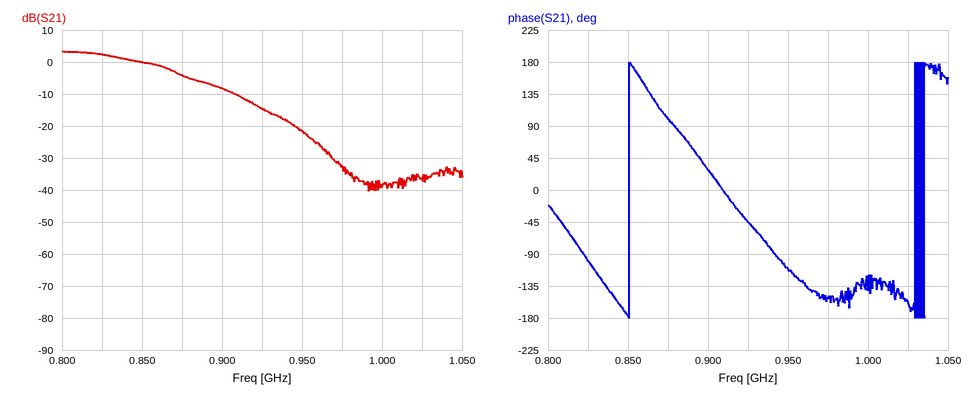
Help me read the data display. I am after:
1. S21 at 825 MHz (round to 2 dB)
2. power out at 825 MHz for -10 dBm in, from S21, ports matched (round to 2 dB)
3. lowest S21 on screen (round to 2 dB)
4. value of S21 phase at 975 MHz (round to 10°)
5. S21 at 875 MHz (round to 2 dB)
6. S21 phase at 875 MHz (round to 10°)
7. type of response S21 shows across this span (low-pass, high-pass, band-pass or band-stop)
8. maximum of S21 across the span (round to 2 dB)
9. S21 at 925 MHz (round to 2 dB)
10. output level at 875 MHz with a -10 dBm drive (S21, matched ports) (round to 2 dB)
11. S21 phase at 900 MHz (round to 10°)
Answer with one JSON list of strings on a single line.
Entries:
["2 dB", "-8 dBm", "-40 dB", "-150°", "-4 dB", "100°", "low-pass", "4 dB", "-14 dB", "-14 dBm", "30°"]
